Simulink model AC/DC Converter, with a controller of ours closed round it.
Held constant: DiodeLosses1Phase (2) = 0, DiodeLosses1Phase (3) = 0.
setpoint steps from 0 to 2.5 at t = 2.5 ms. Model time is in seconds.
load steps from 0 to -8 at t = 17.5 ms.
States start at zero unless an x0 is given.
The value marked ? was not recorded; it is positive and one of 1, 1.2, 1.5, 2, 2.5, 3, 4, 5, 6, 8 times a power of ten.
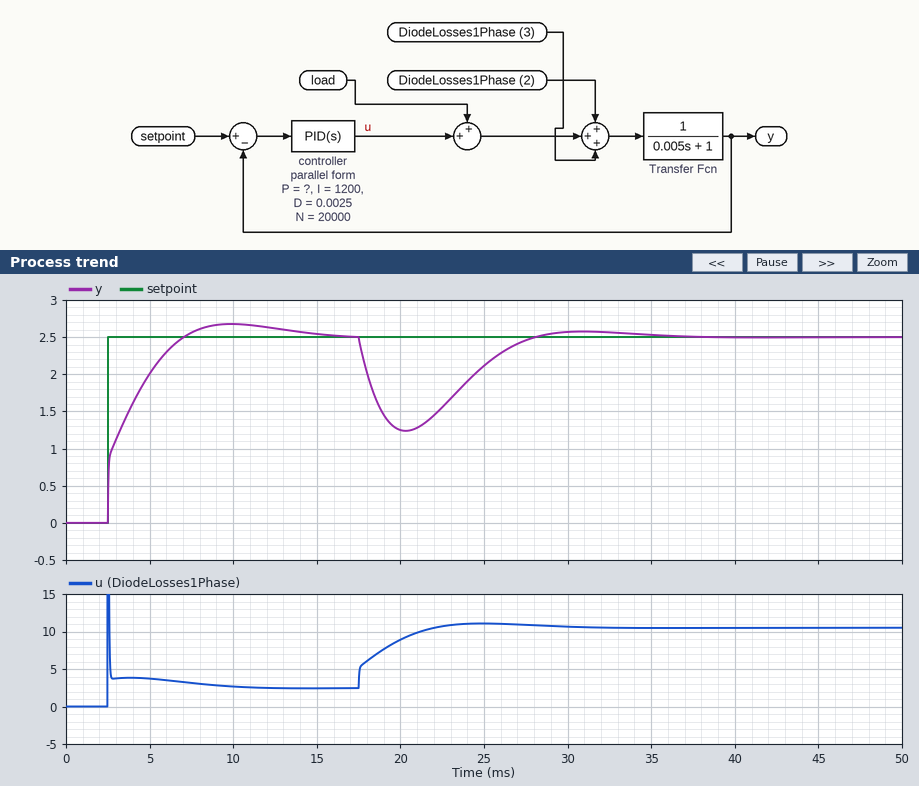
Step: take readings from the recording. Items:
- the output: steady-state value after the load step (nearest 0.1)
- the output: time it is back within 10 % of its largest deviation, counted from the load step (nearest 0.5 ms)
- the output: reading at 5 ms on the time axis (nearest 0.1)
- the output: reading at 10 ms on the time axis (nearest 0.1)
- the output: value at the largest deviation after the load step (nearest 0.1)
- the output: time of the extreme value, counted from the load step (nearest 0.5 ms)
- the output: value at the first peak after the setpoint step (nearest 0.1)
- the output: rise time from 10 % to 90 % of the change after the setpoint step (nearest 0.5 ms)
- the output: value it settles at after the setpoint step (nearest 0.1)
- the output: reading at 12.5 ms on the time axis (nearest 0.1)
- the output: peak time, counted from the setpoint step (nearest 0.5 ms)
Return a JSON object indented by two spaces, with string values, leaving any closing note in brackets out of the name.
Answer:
{
  "the output: steady-state value after the load step": "2.5",
  "the output: time it is back within 10 % of its largest deviation, counted from the load step": "9.0 ms",
  "the output: reading at 5 ms on the time axis": "2.0",
  "the output: reading at 10 ms on the time axis": "2.7",
  "the output: value at the largest deviation after the load step": "1.2",
  "the output: time of the extreme value, counted from the load step": "3.0 ms",
  "the output: value at the first peak after the setpoint step": "2.7",
  "the output: rise time from 10 % to 90 % of the change after the setpoint step": "3.5 ms",
  "the output: value it settles at after the setpoint step": "2.5",
  "the output: reading at 12.5 ms on the time axis": "2.6",
  "the output: peak time, counted from the setpoint step": "7.5 ms"
}
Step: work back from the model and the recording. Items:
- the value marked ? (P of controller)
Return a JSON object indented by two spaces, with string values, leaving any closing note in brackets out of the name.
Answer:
{
  "the value marked ?": "3"
}
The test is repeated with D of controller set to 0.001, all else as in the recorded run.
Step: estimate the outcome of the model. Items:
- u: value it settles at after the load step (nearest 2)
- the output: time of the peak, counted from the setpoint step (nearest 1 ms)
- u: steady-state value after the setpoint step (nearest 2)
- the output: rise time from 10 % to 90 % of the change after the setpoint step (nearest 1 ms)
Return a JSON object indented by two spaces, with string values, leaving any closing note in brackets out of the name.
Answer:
{
  "u: value it settles at after the load step": "10",
  "the output: time of the peak, counted from the setpoint step": "6 ms",
  "u: steady-state value after the setpoint step": "2",
  "the output: rise time from 10 % to 90 % of the change after the setpoint step": "3 ms"
}
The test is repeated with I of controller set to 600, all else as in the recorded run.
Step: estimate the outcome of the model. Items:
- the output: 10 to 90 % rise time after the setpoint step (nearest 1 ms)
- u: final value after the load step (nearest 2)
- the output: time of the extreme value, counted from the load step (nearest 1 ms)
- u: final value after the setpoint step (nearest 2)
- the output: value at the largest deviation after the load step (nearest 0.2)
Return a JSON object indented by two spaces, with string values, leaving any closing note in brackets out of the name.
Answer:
{
  "the output: 10 to 90 % rise time after the setpoint step": "5 ms",
  "u: final value after the load step": "10",
  "the output: time of the extreme value, counted from the load step": "4 ms",
  "u: final value after the setpoint step": "2",
  "the output: value at the largest deviation after the load step": "1.0"
}
